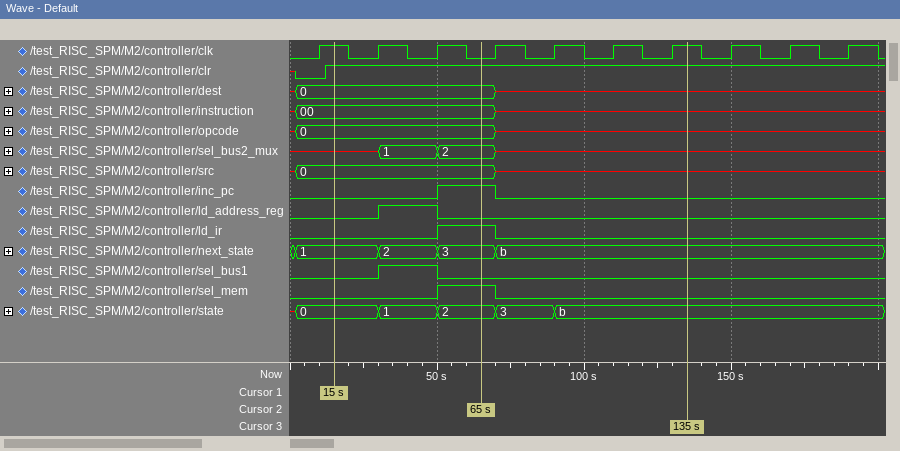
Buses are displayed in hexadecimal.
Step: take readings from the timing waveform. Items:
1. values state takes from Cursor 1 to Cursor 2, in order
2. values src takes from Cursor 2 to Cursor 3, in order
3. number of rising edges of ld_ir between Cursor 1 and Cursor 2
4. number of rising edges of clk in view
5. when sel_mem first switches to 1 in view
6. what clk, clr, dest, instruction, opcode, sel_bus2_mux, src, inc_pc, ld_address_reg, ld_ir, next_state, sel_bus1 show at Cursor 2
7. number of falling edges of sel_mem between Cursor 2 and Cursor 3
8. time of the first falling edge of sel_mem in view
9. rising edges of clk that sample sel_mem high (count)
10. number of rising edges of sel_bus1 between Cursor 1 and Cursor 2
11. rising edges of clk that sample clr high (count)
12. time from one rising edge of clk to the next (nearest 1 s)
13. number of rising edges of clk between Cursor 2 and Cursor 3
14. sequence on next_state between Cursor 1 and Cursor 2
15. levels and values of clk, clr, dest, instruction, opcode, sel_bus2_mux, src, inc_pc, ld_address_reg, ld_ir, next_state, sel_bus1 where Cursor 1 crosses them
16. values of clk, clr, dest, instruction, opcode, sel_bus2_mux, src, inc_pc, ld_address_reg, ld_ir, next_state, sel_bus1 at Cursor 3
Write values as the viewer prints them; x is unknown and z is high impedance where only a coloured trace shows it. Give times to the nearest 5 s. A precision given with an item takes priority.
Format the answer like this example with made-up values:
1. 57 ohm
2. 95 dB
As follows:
1. 0, 1, 2
2. 0, x
3. 1
4. 10
5. 50 s
6. clk=0, clr=1, dest=0, instruction=00, opcode=0, sel_bus2_mux=2, src=0, inc_pc=1, ld_address_reg=0, ld_ir=1, next_state=3, sel_bus1=0
7. 1
8. 70 s
9. 1
10. 1
11. 9
12. 20 s
13. 4
14. 1, 2, 3
15. clk=1, clr=1, dest=0, instruction=00, opcode=0, sel_bus2_mux=x, src=0, inc_pc=0, ld_address_reg=0, ld_ir=0, next_state=1, sel_bus1=0
16. clk=1, clr=1, dest=x, instruction=x, opcode=x, sel_bus2_mux=x, src=x, inc_pc=0, ld_address_reg=0, ld_ir=0, next_state=b, sel_bus1=0
